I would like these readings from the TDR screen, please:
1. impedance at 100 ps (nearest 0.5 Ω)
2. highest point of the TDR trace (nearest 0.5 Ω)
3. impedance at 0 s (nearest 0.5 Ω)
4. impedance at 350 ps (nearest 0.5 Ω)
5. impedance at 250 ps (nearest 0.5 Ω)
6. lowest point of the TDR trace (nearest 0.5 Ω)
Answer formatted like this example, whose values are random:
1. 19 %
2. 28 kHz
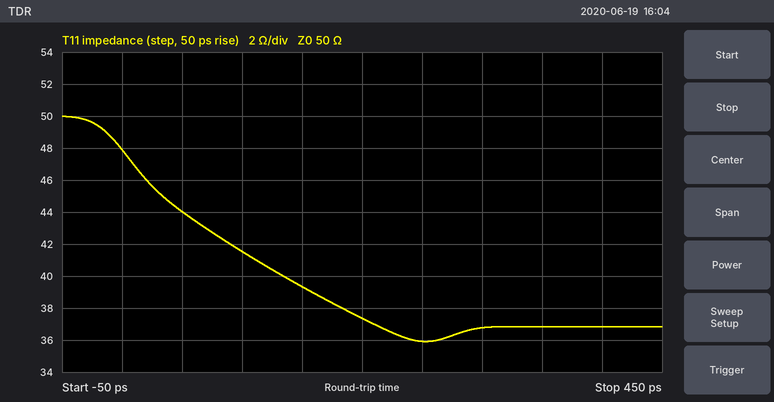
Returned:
1. 41.5 Ω
2. 50.0 Ω
3. 48.0 Ω
4. 37.0 Ω
5. 36.0 Ω
6. 36.0 Ω
